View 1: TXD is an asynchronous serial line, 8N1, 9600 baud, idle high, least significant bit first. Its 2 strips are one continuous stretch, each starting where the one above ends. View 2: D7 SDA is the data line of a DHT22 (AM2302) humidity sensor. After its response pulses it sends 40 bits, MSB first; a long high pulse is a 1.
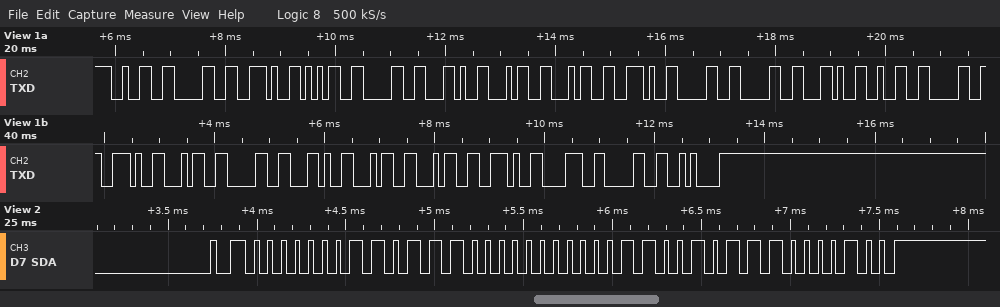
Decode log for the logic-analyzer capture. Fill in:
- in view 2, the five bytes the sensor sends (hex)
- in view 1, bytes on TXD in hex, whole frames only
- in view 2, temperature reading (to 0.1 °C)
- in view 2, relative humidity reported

01 B8 00 CB 84
32 30 2E 35 30 2C 34 34 2E 30 30 2C 32 30 2E 34 30 2C 34 34 2E 38 30 0A
20.3 °C
44.0 %
